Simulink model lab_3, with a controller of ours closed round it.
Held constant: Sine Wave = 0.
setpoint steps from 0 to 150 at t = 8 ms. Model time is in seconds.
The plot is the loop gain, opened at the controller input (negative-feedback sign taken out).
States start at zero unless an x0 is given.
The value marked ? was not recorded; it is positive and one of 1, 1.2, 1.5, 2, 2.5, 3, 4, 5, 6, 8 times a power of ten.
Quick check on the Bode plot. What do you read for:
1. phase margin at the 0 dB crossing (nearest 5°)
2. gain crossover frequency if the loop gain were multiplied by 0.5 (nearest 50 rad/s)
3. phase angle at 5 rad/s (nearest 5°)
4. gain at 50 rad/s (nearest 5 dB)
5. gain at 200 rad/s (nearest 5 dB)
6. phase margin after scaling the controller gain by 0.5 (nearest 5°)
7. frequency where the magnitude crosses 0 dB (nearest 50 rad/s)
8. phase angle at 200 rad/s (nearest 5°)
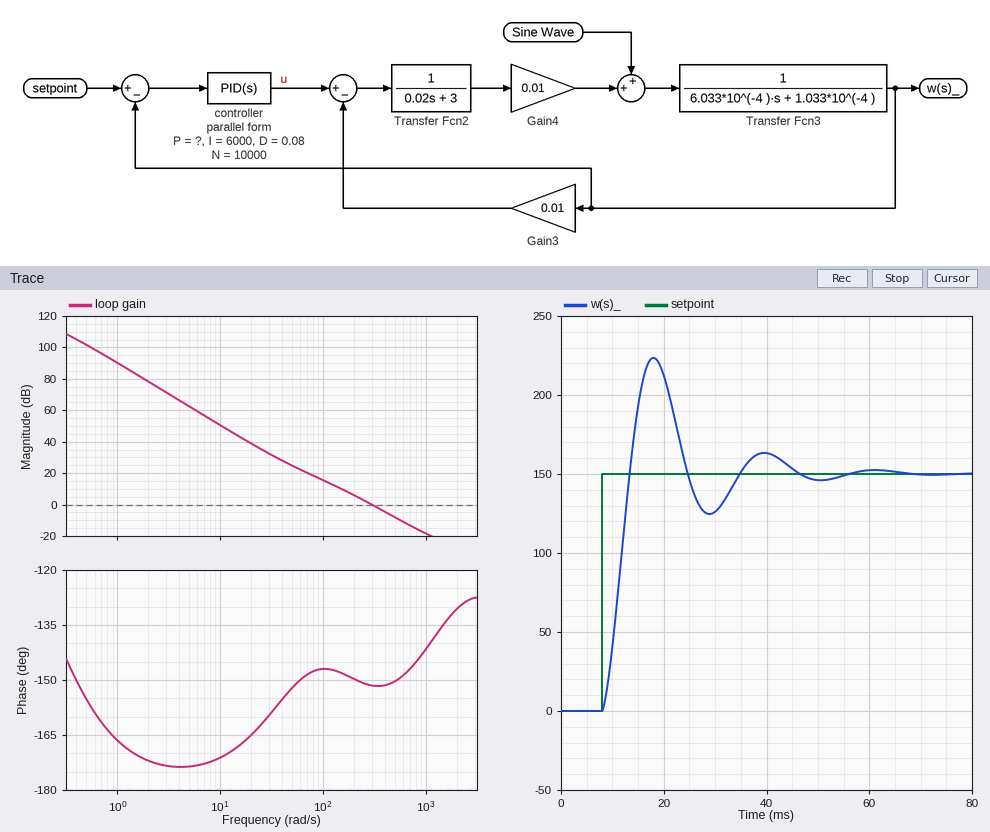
30°
200 rad/s
-175°
25 dB
5 dB
30°
300 rad/s
-150°
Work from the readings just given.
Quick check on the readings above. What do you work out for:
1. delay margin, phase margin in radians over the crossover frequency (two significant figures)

0.0017 s
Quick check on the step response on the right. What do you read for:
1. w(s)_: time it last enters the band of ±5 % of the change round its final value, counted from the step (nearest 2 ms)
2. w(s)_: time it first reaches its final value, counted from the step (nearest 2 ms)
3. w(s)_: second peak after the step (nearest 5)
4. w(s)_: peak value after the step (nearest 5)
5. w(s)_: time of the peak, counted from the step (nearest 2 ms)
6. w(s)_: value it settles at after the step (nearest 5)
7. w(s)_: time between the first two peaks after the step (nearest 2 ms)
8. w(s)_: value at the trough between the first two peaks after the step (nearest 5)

36 ms
6 ms
165
225
10 ms
150
22 ms
125
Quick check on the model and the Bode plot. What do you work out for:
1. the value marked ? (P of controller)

120
